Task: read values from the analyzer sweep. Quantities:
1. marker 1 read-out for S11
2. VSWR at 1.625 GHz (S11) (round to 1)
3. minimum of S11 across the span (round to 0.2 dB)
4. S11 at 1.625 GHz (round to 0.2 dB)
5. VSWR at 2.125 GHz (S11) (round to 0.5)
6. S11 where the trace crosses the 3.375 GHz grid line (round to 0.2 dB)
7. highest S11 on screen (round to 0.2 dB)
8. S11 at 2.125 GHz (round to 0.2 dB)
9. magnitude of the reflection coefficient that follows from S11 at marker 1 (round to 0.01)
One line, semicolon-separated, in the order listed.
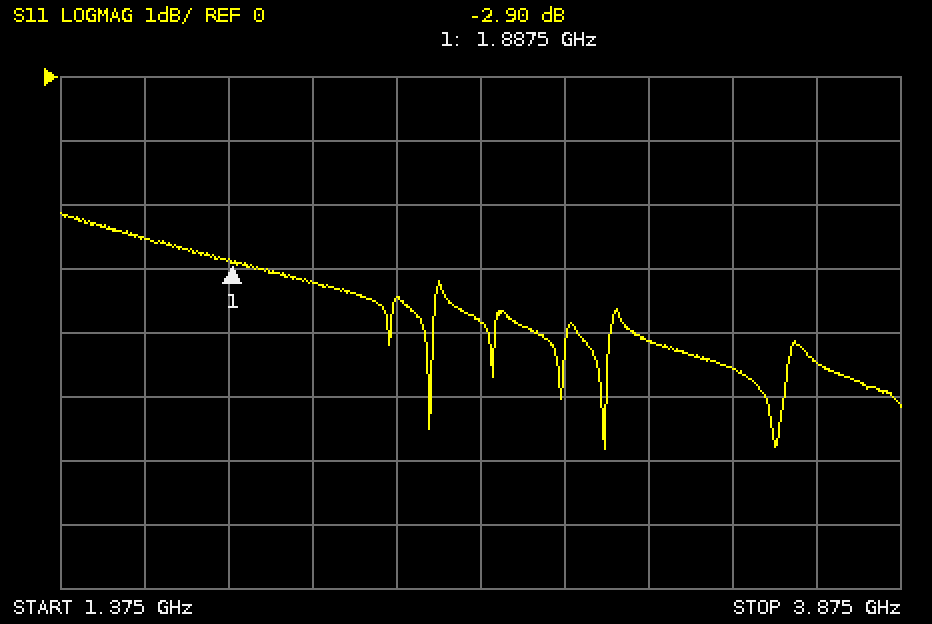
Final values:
-2.90 dB; 7; -5.8 dB; -2.6 dB; 5.5; -4.6 dB; -2.2 dB; -3.2 dB; 0.72
